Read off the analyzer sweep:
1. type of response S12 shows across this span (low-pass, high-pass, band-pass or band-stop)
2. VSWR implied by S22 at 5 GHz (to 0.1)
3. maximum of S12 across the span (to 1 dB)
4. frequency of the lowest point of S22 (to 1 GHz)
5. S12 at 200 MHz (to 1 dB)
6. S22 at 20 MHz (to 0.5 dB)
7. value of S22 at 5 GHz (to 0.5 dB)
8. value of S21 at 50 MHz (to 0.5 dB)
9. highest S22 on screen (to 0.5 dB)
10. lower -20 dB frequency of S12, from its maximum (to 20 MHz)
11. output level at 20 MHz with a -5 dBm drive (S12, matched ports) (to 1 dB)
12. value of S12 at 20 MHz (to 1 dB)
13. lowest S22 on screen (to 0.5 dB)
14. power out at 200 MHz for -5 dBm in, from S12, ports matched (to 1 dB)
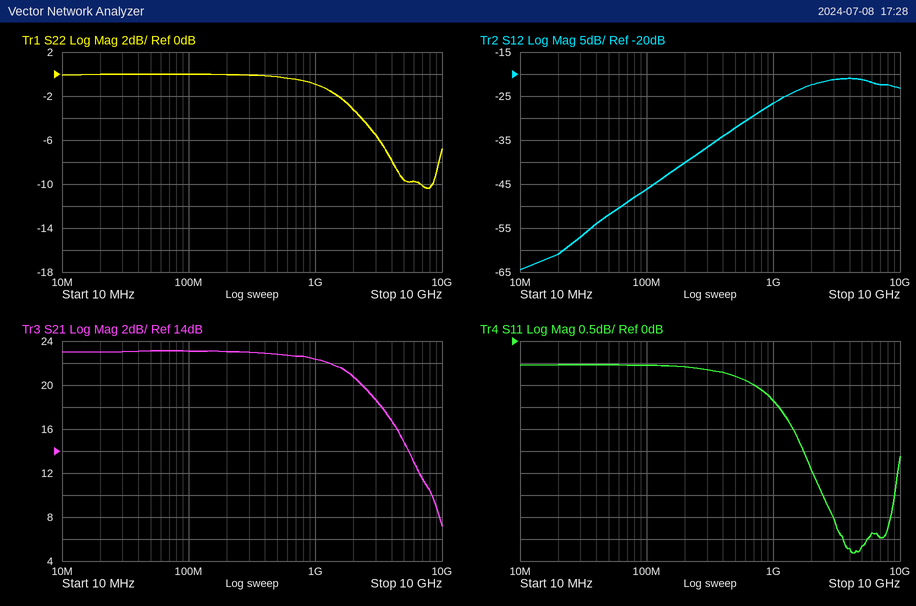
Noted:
high-pass
2.0
-21 dB
8 GHz
-40 dB
0.0 dB
-9.5 dB
23.0 dB
0.0 dB
180 MHz
-66 dBm
-61 dB
-10.5 dB
-45 dBm
